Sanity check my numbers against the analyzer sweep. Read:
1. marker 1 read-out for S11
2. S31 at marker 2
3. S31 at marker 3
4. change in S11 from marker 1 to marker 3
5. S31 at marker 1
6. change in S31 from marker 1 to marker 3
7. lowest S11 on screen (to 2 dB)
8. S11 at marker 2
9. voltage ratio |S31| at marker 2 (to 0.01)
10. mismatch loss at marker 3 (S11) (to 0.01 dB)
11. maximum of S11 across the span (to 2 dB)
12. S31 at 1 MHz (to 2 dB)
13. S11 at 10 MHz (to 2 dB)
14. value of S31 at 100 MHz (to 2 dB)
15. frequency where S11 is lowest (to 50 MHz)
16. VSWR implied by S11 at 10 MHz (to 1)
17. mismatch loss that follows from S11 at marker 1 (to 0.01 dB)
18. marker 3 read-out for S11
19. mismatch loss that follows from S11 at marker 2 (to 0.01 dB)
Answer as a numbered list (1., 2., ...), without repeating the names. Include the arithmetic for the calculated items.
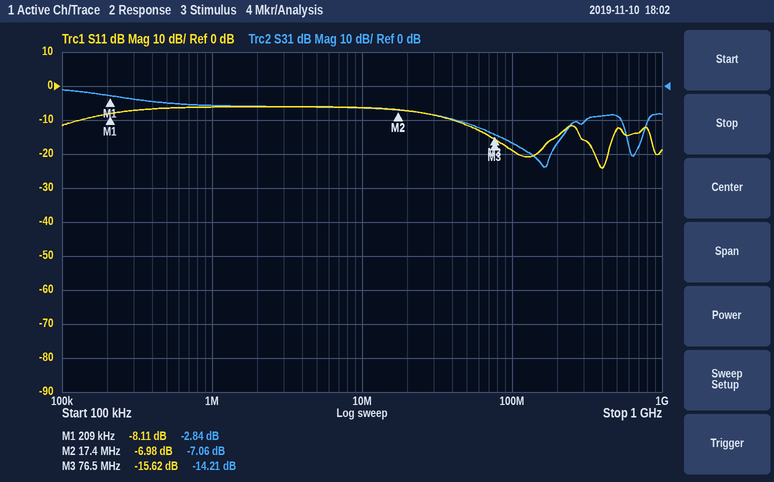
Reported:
1. -8.11 dB
2. -7.06 dB
3. -14.21 dB
4. -15.62 − (-8.11) = -7.51 dB
5. -2.84 dB
6. -14.21 − (-2.84) = -11.37 dB
7. -24 dB
8. -6.98 dB
9. 10^(-7.06/20) ≈ 0.44
10. −10 log10(1 − 10^(-15.62/10)) ≈ 0.12 dB
11. -6 dB
12. -6 dB
13. -6 dB
14. -16 dB
15. 400 MHz
16. |Γ| = 10^(-6/20) = 0.5012; VSWR = (1 + 0.5012)/(1 − 0.5012) ≈ 3
17. −10 log10(1 − 10^(-8.11/10)) ≈ 0.73 dB
18. -15.62 dB
19. −10 log10(1 − 10^(-6.98/10)) ≈ 0.97 dB
